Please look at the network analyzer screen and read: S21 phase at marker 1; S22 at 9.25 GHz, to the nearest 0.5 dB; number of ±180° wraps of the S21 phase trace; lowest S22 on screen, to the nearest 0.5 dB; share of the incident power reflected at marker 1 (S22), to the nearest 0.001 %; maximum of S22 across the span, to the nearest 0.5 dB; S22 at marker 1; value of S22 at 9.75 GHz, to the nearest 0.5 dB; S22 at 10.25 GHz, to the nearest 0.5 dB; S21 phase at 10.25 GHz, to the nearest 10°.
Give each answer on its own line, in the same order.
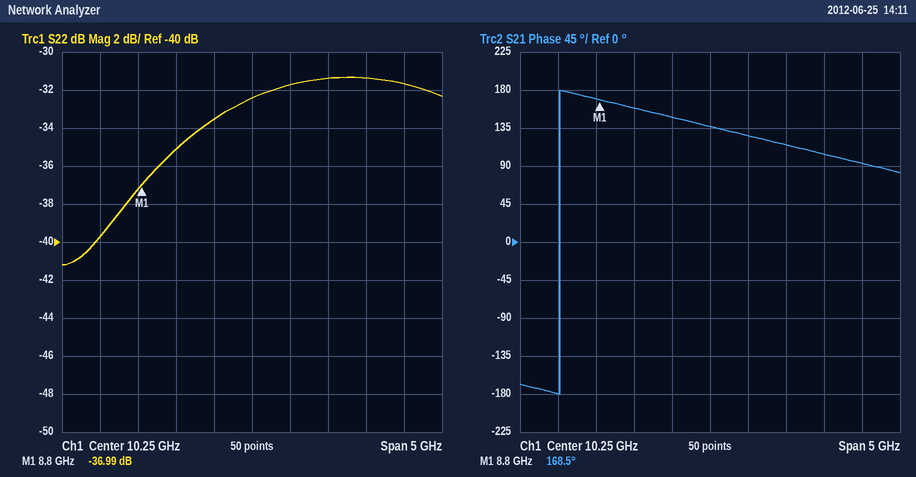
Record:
168.5°
-35.0 dB
1
-41.0 dB
0.020 %
-31.5 dB
-36.99 dB
-33.5 dB
-32.5 dB
140°
